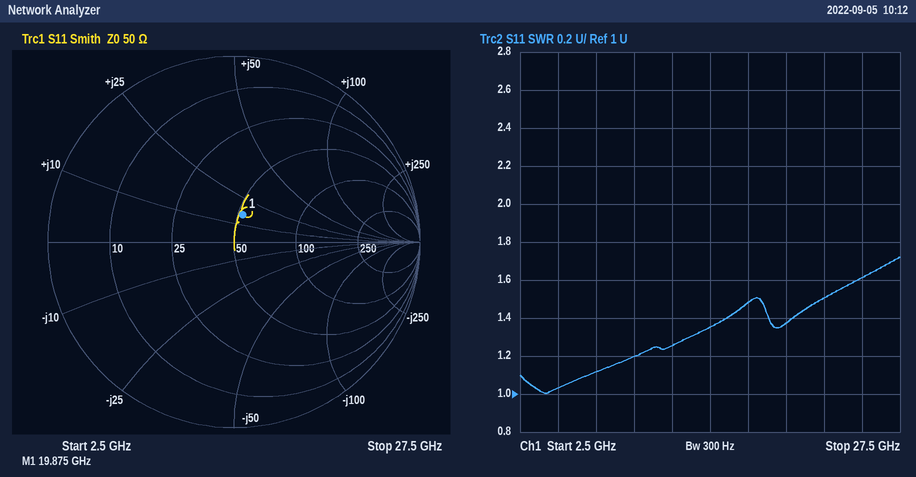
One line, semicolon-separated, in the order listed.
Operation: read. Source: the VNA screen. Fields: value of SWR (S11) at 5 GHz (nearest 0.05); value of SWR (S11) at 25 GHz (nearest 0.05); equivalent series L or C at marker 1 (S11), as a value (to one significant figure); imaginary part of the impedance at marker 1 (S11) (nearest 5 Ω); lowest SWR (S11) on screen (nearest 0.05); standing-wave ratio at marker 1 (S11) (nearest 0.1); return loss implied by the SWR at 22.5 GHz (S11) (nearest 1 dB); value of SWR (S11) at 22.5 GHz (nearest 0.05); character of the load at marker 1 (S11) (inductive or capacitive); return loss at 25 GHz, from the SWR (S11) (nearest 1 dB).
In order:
1.05; 1.60; 100 pH; +15 Ω; 1.00; 1.4; 14 dB; 1.50; inductive; 13 dB
